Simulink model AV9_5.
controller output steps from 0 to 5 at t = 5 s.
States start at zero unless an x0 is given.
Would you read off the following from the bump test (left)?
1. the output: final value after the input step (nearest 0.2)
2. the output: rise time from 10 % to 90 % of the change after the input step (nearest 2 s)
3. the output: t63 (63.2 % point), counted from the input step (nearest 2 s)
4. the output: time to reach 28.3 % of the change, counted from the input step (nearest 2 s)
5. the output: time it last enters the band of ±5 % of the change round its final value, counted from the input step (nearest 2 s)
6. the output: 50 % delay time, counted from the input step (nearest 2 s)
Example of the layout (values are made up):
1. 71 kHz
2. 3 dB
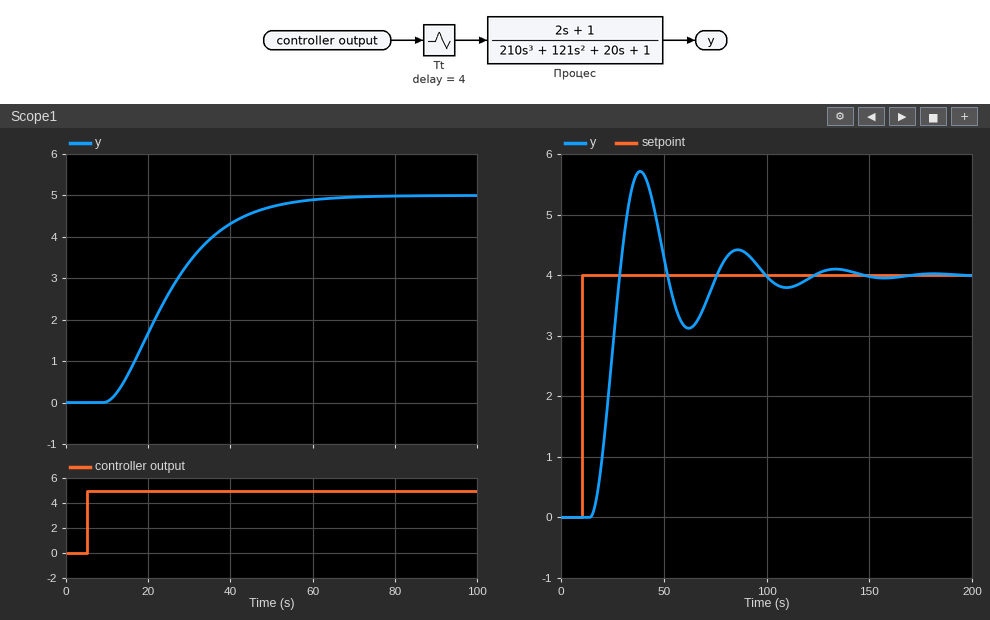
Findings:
1. 5.0
2. 30 s
3. 24 s
4. 14 s
5. 46 s
6. 20 s
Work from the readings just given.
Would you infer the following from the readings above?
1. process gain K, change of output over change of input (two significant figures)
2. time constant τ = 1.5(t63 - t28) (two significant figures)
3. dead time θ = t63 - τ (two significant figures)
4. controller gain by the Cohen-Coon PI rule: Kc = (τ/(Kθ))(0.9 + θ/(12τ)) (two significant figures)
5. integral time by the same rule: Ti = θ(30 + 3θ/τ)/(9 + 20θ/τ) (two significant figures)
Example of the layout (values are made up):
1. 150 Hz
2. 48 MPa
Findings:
1. 1.0
2. 15 s
3. 9.0 s
4. 1.6
5. 14 s
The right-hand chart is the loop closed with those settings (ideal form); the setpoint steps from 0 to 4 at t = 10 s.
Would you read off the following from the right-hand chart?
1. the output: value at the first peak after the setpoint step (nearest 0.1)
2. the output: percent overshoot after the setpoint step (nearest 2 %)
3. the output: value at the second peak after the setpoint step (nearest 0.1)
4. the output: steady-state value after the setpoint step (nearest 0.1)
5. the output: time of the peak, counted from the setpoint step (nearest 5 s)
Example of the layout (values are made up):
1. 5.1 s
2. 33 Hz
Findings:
1. 5.7
2. 42 %
3. 4.4
4. 4.0
5. 30 s
